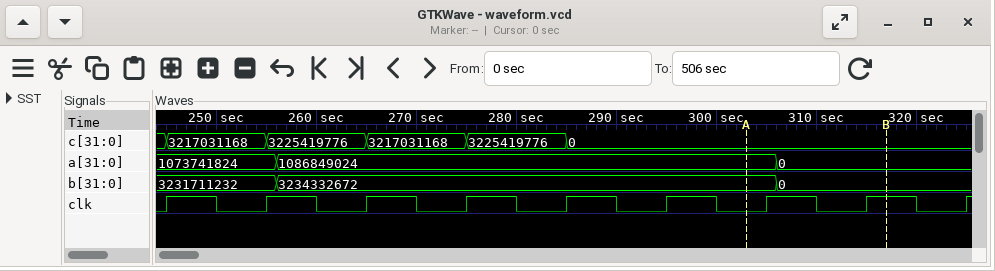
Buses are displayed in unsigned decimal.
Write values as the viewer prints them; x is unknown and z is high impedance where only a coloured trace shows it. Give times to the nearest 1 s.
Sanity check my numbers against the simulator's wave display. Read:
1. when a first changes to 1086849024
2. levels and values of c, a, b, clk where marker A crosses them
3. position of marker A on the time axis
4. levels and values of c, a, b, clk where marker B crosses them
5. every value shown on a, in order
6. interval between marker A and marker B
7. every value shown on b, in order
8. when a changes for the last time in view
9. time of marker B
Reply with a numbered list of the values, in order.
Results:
1. 256 s
2. c=0, a=1086849024, b=3234332672, clk=0
3. 303 s
4. c=0, a=0, b=0, clk=1
5. 1073741824, 1086849024, 0
6. 14 s
7. 3231711232, 3234332672, 0
8. 306 s
9. 317 s
